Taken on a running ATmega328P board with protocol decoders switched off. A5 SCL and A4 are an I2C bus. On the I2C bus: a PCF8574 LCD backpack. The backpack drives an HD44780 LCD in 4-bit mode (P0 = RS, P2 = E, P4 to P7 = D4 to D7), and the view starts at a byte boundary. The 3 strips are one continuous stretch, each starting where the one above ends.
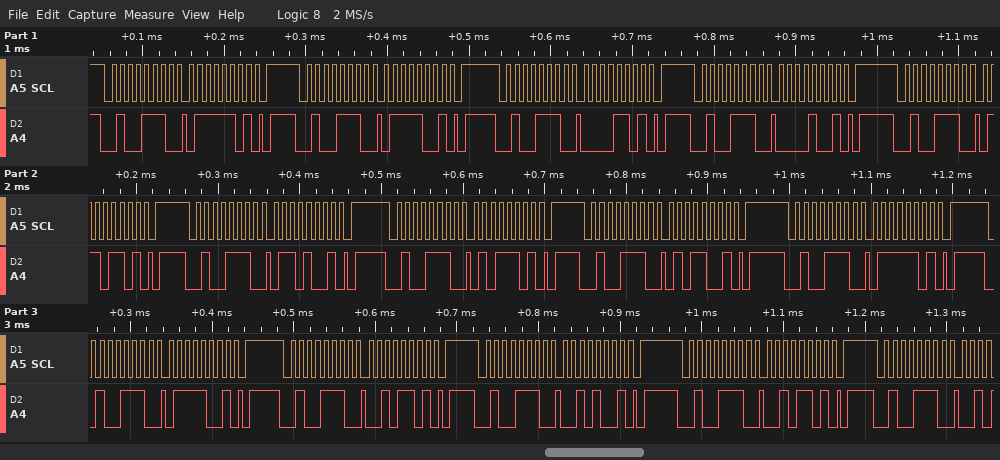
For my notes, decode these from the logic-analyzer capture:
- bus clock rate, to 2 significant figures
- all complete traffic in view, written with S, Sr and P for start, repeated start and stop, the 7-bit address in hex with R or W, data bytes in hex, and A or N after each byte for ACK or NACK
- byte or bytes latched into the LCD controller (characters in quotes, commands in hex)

100 kHz
S 27W A 7D A P S 27W A 79 A P S 27W A 0D A P S 27W A 09 A P S 27W A 6D A P S 27W A 69 A P S 27W A 5D A P S 27W A 59 A P S 27W A 7D A P S 27W A 79 A P S 27W A 2D A P S 27W A 29 A P S 27W A 2D A P S 27W A
'p' 'e' 'r'
